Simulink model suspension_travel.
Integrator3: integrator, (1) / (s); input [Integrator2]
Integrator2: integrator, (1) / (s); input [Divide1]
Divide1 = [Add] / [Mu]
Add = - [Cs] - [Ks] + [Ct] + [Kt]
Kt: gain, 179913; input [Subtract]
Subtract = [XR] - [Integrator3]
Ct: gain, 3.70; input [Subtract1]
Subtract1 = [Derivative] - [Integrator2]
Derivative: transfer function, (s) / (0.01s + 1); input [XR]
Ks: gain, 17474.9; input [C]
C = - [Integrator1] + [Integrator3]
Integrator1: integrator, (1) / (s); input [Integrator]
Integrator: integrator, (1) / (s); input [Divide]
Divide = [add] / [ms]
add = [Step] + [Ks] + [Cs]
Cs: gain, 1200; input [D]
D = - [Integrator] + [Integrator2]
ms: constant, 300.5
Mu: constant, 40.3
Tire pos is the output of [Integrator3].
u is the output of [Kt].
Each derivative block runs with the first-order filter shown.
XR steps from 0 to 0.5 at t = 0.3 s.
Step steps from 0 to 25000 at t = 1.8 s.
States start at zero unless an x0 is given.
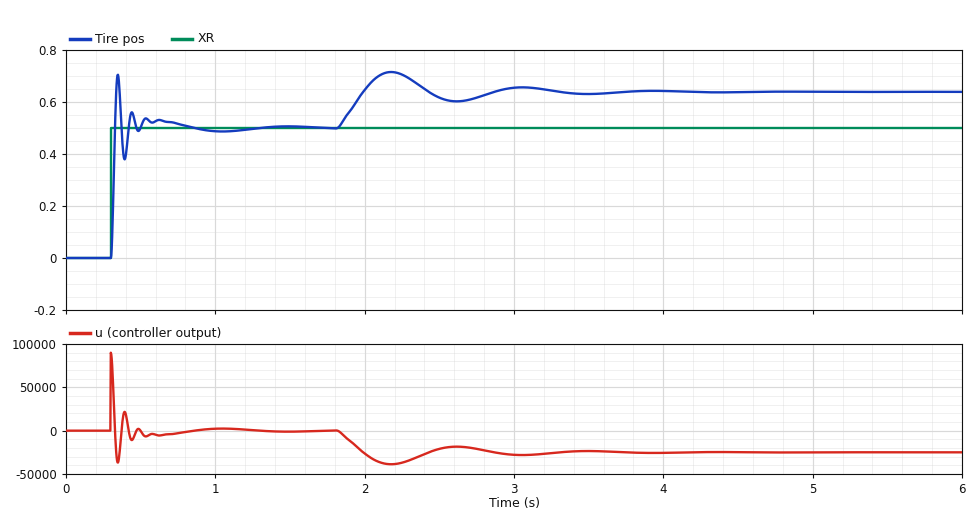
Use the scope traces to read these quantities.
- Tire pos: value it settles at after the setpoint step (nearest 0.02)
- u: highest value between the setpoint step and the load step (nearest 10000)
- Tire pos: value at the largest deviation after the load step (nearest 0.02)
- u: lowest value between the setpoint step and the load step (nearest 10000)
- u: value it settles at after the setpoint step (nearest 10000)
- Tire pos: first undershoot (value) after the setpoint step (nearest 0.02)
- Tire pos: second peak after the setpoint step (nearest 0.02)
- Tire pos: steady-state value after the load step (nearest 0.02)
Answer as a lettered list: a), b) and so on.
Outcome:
a) 0.50
b) 90000
c) 0.72
d) -40000
e) 0
f) 0.38
g) 0.56
h) 0.64
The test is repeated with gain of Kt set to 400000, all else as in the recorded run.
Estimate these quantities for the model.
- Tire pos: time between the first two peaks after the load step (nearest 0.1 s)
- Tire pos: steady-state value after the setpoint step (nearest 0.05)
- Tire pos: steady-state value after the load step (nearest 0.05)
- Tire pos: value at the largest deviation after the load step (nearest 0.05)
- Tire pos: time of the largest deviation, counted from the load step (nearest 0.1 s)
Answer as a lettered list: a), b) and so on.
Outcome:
a) 0.9 s
b) 0.50
c) 0.55
d) 0.60
e) 0.4 s
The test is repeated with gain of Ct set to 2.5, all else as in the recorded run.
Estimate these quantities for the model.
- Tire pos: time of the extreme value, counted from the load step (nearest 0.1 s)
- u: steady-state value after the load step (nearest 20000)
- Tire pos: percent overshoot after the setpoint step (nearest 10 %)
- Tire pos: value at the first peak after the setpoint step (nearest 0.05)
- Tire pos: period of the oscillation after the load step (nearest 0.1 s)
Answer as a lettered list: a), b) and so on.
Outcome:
a) 0.4 s
b) -20000
c) 40 %
d) 0.70
e) 0.9 s
